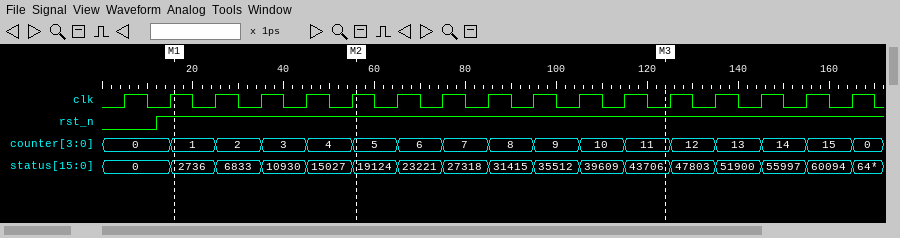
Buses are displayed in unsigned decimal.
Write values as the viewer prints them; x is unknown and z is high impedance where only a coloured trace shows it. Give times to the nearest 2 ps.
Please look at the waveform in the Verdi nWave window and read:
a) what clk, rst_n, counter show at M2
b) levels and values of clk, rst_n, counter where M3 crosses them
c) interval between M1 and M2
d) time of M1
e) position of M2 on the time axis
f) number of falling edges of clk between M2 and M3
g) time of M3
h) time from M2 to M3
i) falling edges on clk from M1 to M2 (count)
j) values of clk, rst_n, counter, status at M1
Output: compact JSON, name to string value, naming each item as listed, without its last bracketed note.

{"what clk, rst_n, counter show at M2": "clk=1, rst_n=1, counter=5", "levels and values of clk, rst_n, counter where M3 crosses them": "clk=0, rst_n=1, counter=11", "interval between M1 and M2": "40 ps", "time of M1": "16 ps", "position of M2 on the time axis": "56 ps", "number of falling edges of clk between M2 and M3": "7", "time of M3": "124 ps", "time from M2 to M3": "68 ps", "falling edges on clk from M1 to M2": "4", "values of clk, rst_n, counter, status at M1": "clk=1, rst_n=1, counter=1, status=2736"}
